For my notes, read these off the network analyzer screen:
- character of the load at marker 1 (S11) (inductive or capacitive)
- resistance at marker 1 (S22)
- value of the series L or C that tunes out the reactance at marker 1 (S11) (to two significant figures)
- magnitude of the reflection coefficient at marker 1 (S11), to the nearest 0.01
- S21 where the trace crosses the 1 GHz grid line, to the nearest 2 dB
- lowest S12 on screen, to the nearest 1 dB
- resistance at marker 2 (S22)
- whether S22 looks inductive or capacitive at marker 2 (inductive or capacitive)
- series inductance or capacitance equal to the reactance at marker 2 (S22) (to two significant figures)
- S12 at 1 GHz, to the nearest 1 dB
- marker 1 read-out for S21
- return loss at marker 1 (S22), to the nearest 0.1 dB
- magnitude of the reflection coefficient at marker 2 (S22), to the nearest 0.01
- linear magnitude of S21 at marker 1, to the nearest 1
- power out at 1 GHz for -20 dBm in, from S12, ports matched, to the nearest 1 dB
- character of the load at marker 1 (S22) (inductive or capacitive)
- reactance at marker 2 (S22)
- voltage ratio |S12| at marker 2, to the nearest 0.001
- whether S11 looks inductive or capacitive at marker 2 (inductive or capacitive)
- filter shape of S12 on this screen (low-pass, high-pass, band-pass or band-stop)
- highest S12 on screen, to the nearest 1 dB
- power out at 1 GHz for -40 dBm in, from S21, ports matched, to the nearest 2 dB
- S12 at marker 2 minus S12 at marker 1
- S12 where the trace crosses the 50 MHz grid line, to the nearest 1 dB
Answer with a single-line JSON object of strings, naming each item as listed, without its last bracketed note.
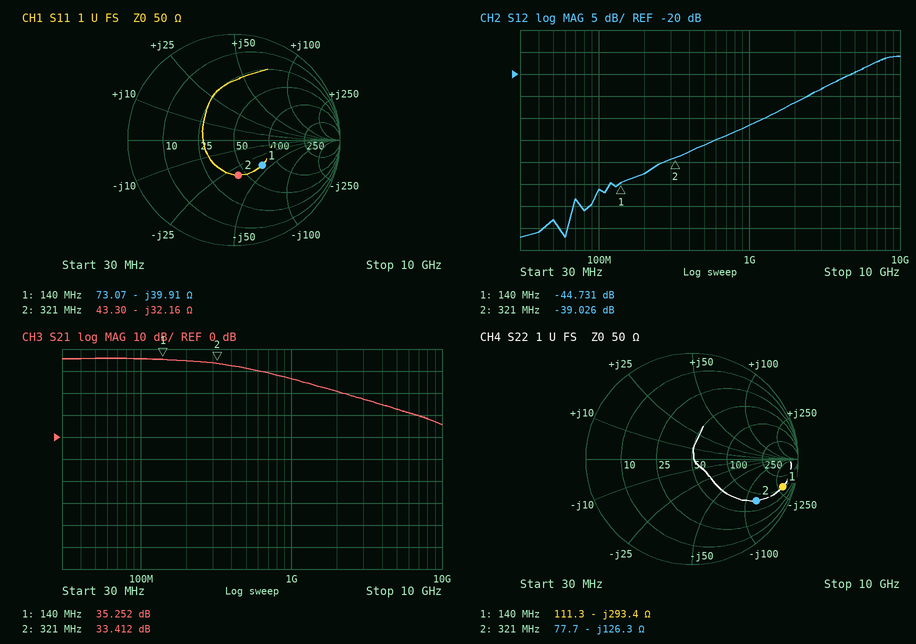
{"character of the load at marker 1 (S11)": "capacitive", "resistance at marker 1": "111.3 Ω", "value of the series L or C that tunes out the reactance at marker 1 (S11)": "45 nH", "magnitude of the reflection coefficient at marker 1 (S11), to the nearest 0.01": "0.36", "S21 where the trace crosses the 1 GHz grid line, to the nearest 2 dB": "26 dB", "lowest S12 on screen, to the nearest 1 dB": "-57 dB", "resistance at marker 2": "77.7 Ω", "whether S22 looks inductive or capacitive at marker 2": "capacitive", "series inductance or capacitance equal to the reactance at marker 2 (S22)": "3.9 pF", "S12 at 1 GHz, to the nearest 1 dB": "-32 dB", "marker 1 read-out for S21": "35.252 dB", "return loss at marker 1 (S22), to the nearest 0.1 dB": "1.0 dB", "magnitude of the reflection coefficient at marker 2 (S22), to the nearest 0.01": "0.72", "linear magnitude of S21 at marker 1, to the nearest 1": "58", "power out at 1 GHz for -20 dBm in, from S12, ports matched, to the nearest 1 dB": "-52 dBm", "character of the load at marker 1 (S22)": "capacitive", "reactance at marker 2": "-126.3 Ω", "voltage ratio |S12| at marker 2, to the nearest 0.001": "0.011", "whether S11 looks inductive or capacitive at marker 2": "capacitive", "filter shape of S12 on this screen": "high-pass", "highest S12 on screen, to the nearest 1 dB": "-16 dB", "power out at 1 GHz for -40 dBm in, from S21, ports matched, to the nearest 2 dB": "-14 dBm", "S12 at marker 2 minus S12 at marker 1": "5.705 dB", "S12 where the trace crosses the 50 MHz grid line, to the nearest 1 dB": "-53 dB"}
